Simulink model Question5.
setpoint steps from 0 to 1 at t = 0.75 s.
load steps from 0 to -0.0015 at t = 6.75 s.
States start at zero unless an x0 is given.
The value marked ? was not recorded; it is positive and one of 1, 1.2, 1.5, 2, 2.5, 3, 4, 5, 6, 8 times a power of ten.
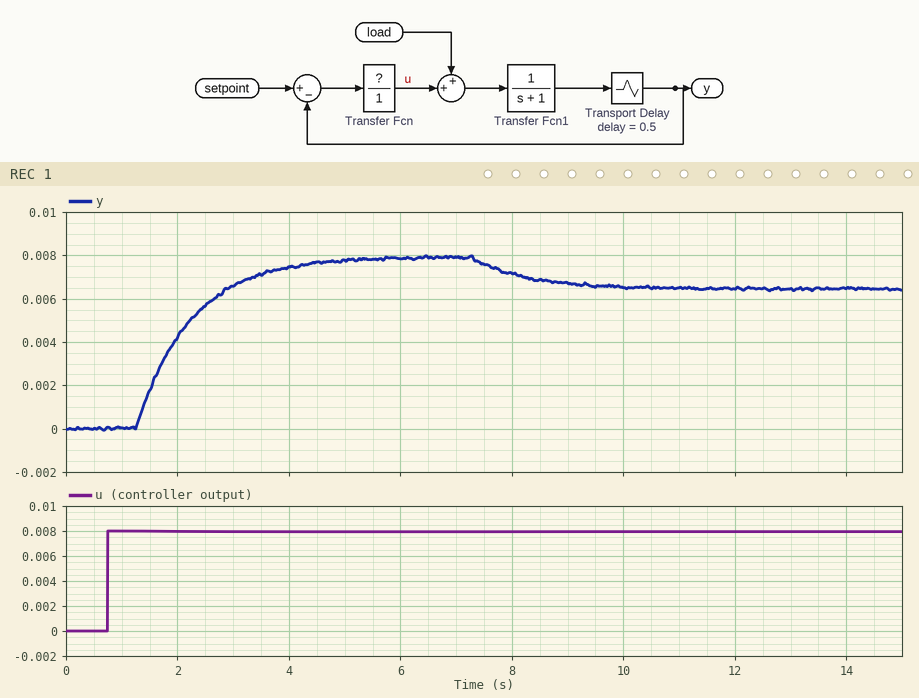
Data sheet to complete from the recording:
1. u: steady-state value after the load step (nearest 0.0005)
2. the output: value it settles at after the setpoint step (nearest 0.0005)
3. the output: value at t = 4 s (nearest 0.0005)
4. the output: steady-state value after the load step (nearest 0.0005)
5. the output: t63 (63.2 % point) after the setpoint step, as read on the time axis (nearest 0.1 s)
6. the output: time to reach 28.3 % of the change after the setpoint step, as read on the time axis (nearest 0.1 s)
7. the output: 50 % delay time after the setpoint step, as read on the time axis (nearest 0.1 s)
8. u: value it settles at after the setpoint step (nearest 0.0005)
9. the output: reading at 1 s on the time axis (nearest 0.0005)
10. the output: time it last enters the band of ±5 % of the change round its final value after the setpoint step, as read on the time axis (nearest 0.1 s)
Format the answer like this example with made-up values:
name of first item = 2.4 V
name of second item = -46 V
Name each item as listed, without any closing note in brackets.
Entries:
u: steady-state value after the load step = 0.0080
the output: value it settles at after the setpoint step = 0.0080
the output: value at t = 4 s = 0.0075
the output: steady-state value after the load step = 0.0065
the output: t63 (63.2 % point) after the setpoint step, as read on the time axis = 2.2 s
the output: time to reach 28.3 % of the change after the setpoint step, as read on the time axis = 1.6 s
the output: 50 % delay time after the setpoint step, as read on the time axis = 1.9 s
u: value it settles at after the setpoint step = 0.0080
the output: reading at 1 s on the time axis = 0.0000
the output: time it last enters the band of ±5 % of the change round its final value after the setpoint step, as read on the time axis = 4.2 s
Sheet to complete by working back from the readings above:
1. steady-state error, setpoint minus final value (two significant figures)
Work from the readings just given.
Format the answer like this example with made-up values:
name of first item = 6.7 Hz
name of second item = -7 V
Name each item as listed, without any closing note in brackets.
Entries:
steady-state error, setpoint minus final value = 0.99
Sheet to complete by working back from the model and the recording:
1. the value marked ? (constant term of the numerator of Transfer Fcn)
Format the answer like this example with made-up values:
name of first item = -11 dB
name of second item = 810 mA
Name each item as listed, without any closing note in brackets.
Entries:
the value marked ? = 0.008
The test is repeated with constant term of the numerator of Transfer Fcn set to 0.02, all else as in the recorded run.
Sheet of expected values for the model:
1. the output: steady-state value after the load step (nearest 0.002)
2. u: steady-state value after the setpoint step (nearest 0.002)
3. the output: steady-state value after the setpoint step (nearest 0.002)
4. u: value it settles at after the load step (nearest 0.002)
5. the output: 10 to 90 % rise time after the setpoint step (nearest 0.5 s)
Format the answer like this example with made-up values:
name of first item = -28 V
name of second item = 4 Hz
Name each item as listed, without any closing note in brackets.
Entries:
the output: steady-state value after the load step = 0.018
u: steady-state value after the setpoint step = 0.020
the output: steady-state value after the setpoint step = 0.020
u: value it settles at after the load step = 0.020
the output: 10 to 90 % rise time after the setpoint step = 2.0 s
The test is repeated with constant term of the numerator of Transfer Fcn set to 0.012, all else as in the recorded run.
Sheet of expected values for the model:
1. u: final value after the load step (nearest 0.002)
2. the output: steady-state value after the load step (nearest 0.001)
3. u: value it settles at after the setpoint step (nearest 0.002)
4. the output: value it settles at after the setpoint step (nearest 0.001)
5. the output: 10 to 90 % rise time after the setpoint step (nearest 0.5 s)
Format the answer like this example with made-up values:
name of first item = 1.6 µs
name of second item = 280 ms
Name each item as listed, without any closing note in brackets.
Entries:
u: final value after the load step = 0.012
the output: steady-state value after the load step = 0.010
u: value it settles at after the setpoint step = 0.012
the output: value it settles at after the setpoint step = 0.012
the output: 10 to 90 % rise time after the setpoint step = 2.0 s
